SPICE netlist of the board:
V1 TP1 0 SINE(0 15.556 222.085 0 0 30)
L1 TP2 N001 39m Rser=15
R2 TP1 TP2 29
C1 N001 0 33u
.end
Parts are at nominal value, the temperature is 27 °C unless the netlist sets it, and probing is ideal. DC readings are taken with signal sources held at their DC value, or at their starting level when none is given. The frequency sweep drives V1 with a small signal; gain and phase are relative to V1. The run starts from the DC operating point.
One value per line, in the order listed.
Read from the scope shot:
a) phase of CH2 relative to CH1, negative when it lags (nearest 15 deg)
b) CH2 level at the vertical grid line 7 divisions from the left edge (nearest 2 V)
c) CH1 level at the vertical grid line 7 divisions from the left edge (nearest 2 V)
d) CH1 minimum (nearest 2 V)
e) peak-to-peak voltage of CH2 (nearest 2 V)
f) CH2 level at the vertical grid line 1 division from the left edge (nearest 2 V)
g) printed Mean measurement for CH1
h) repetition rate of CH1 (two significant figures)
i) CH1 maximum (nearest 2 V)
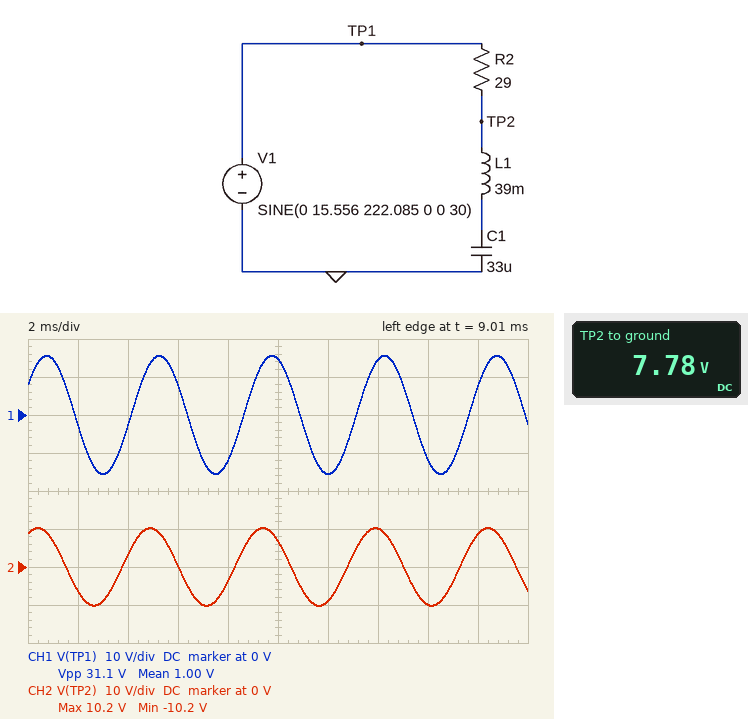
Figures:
30 deg
10 V
14 V
-16 V
20 V
-6 V
1.00 V
220 Hz
16 V
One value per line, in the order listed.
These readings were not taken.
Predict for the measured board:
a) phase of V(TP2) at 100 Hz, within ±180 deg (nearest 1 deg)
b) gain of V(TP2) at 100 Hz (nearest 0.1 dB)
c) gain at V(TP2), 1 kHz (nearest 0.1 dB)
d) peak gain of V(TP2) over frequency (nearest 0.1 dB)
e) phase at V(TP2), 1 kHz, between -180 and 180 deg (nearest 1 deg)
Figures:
-29 deg
-5.0 dB
-0.1 dB
0 dB
7 deg
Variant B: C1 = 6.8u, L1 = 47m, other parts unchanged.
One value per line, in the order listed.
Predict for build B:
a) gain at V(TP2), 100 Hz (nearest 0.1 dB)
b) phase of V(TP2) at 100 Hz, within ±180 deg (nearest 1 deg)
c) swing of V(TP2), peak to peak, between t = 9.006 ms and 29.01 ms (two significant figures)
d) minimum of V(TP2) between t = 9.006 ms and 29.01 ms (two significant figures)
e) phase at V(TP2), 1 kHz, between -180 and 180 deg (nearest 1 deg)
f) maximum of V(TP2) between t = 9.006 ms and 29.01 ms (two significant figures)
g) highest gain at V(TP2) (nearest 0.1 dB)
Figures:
-0.2 dB
-8 deg
22 V
-11 V
6 deg
11 V
0 dB
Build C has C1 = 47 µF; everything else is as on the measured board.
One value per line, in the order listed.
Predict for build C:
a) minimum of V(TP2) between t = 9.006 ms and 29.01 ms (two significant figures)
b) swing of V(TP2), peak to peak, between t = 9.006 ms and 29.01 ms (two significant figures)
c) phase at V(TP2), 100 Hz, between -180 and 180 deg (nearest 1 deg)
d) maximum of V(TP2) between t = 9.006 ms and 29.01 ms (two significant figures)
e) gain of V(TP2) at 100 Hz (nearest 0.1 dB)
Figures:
-11 V
22 V
-20 deg
11 V
-8.1 dB
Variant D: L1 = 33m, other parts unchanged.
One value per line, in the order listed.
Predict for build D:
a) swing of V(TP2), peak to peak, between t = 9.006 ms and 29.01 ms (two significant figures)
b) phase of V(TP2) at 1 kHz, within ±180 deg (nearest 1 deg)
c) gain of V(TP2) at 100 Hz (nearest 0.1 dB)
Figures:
18 V
8 deg
-4.4 dB
